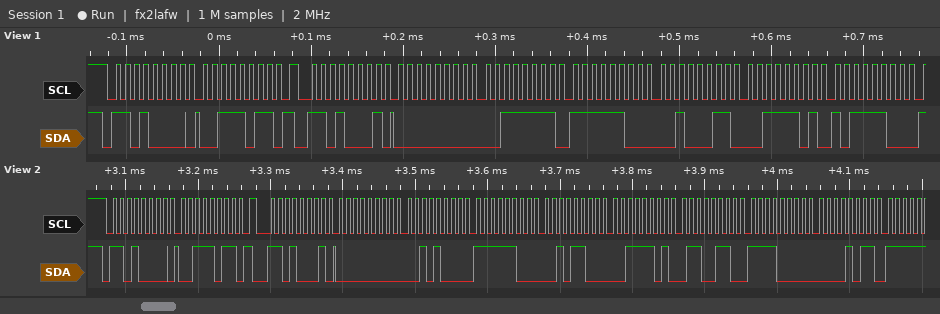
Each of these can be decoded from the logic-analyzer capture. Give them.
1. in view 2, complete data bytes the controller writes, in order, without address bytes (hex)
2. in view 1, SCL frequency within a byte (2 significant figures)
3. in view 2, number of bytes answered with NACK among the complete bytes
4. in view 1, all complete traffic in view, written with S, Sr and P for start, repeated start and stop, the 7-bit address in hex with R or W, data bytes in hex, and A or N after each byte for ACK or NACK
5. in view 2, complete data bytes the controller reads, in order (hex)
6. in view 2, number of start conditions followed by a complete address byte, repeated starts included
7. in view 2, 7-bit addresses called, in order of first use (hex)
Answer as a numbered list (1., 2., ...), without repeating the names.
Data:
1. 3B
2. 100 kHz
3. 0
4. S 68W A 3B A Sr 68R A 00 A 3F A FC A 23 A 3D A BC A
5. 00 28 FC 2C 3D 66 F0 0B
6. 2
7. 0x68
